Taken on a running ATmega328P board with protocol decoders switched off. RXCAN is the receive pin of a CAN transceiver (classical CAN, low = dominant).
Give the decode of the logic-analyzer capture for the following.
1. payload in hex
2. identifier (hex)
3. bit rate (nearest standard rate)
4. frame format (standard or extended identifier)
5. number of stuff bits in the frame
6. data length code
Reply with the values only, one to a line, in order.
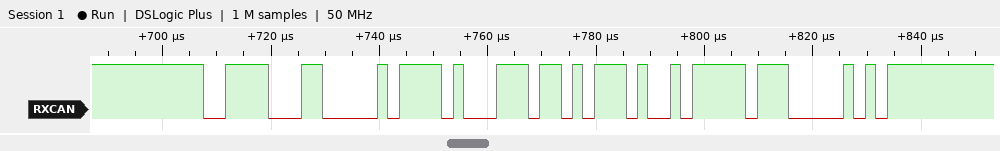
D1 DA E9
0x3C6
500 kbit/s
standard
3
3
